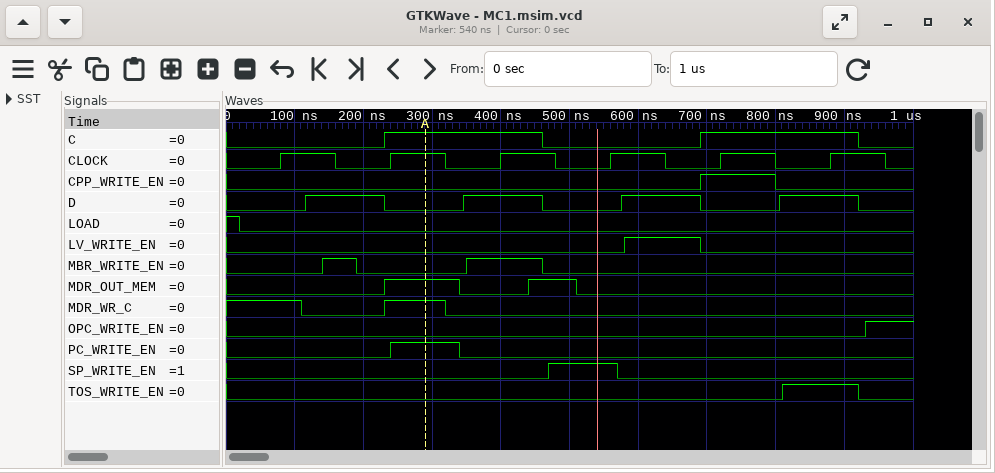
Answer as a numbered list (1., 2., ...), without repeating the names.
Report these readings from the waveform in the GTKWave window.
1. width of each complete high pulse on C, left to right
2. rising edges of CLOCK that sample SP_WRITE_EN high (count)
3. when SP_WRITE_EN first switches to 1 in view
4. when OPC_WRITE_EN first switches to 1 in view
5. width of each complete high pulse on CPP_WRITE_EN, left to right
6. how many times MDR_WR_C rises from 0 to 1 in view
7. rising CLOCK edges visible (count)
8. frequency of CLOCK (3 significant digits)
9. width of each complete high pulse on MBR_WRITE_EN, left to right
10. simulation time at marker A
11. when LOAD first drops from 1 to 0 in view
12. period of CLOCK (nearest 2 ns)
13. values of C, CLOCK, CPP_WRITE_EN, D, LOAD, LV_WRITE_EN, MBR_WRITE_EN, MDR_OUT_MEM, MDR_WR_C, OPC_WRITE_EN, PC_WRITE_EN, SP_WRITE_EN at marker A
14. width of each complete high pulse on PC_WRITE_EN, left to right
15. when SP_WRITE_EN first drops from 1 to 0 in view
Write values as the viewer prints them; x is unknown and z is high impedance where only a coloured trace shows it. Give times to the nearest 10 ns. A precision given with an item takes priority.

1. 230 ns, 230 ns
2. 1
3. 470 ns
4. 930 ns
5. 110 ns
6. 1
7. 6
8. 6.25 MHz
9. 50 ns, 110 ns
10. 290 ns
11. 20 ns
12. 160 ns
13. C=1, CLOCK=1, CPP_WRITE_EN=0, D=0, LOAD=0, LV_WRITE_EN=0, MBR_WRITE_EN=0, MDR_OUT_MEM=1, MDR_WR_C=1, OPC_WRITE_EN=0, PC_WRITE_EN=1, SP_WRITE_EN=0
14. 100 ns
15. 570 ns
